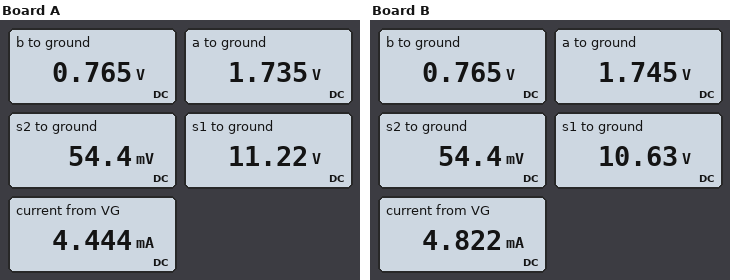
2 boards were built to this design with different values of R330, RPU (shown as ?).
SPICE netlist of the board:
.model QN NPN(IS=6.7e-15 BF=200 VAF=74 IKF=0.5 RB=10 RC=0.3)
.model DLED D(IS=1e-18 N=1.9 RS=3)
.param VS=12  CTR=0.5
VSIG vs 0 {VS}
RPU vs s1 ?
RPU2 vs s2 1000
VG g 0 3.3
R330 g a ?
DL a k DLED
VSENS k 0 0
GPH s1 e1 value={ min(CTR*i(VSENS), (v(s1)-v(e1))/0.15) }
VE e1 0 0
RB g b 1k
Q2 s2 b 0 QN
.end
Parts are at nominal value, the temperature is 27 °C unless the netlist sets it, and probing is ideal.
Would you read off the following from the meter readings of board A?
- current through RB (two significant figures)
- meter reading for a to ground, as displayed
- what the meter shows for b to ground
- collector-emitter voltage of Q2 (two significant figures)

2.5 mA
1.735 V
0.765 V
54 mV
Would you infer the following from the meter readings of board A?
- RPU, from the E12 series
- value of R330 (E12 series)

820 Ω
820 Ω
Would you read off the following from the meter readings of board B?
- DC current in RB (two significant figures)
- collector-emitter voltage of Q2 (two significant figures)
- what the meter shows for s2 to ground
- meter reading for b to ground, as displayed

2.5 mA
54 mV
54.4 mV
0.765 V
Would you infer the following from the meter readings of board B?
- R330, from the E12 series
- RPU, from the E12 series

680 Ω
1.2 kΩ
